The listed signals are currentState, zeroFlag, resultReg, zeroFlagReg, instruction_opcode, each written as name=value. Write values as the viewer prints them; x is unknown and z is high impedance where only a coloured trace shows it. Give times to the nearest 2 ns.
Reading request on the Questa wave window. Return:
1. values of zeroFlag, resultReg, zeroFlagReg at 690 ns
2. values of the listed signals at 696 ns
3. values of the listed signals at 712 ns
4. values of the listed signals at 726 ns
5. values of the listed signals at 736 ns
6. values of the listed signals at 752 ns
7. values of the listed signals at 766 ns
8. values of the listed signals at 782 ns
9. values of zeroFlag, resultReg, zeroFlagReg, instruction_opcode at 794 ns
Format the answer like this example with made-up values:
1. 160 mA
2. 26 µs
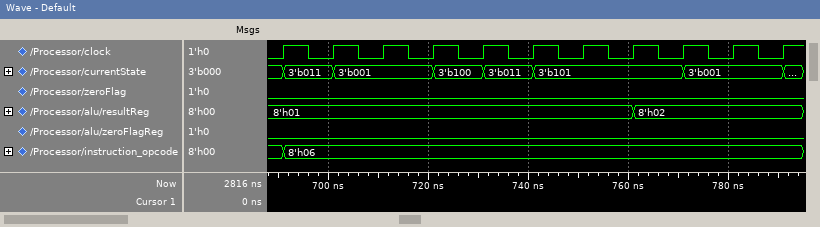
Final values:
1. zeroFlag=0, resultReg=8'h01, zeroFlagReg=0
2. currentState=3'b011, zeroFlag=0, resultReg=8'h01, zeroFlagReg=0, instruction_opcode=8'h06
3. currentState=3'b001, zeroFlag=0, resultReg=8'h01, zeroFlagReg=0, instruction_opcode=8'h06
4. currentState=3'b100, zeroFlag=0, resultReg=8'h01, zeroFlagReg=0, instruction_opcode=8'h06
5. currentState=3'b011, zeroFlag=0, resultReg=8'h01, zeroFlagReg=0, instruction_opcode=8'h06
6. currentState=3'b101, zeroFlag=0, resultReg=8'h01, zeroFlagReg=0, instruction_opcode=8'h06
7. currentState=3'b101, zeroFlag=0, resultReg=8'h02, zeroFlagReg=0, instruction_opcode=8'h06
8. currentState=3'b001, zeroFlag=0, resultReg=8'h02, zeroFlagReg=0, instruction_opcode=8'h06
9. zeroFlag=0, resultReg=8'h02, zeroFlagReg=0, instruction_opcode=8'h06
